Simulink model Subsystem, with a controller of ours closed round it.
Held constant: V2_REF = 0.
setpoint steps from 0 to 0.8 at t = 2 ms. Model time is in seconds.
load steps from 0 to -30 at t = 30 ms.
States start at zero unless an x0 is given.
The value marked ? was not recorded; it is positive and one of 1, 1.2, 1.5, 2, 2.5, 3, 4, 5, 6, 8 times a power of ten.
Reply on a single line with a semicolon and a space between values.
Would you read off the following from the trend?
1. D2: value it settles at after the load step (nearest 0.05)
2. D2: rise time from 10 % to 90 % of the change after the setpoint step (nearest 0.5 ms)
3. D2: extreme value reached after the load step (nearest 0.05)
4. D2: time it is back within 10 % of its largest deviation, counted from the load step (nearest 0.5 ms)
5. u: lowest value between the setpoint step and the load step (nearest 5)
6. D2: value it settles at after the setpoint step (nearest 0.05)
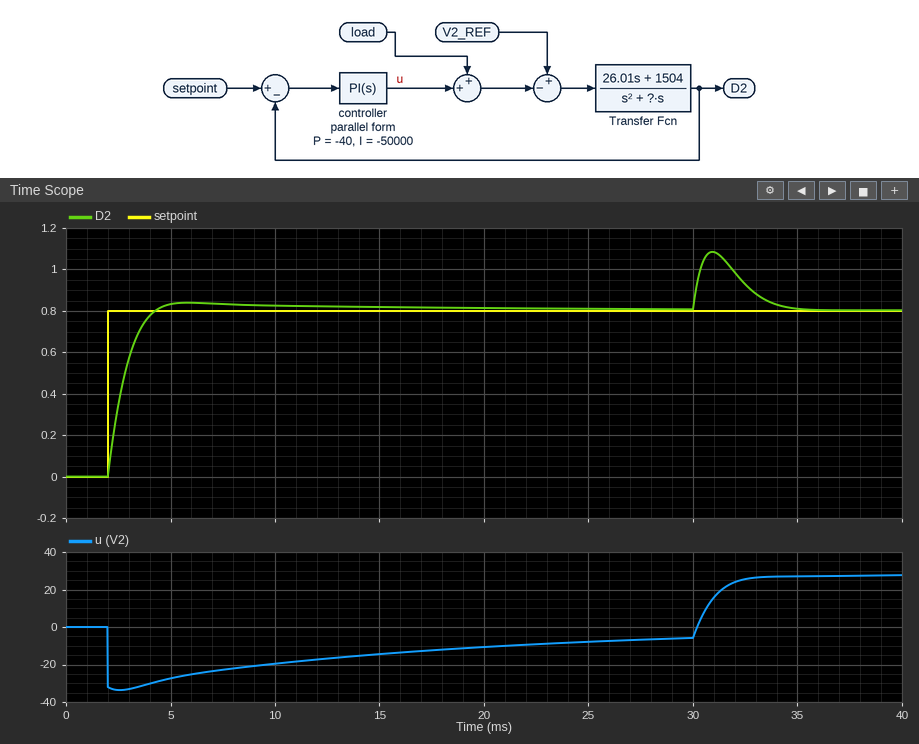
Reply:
0.80; 1.5 ms; 1.10; 4.0 ms; -35; 0.80
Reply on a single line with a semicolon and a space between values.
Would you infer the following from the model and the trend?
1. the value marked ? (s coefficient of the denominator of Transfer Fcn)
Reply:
1000
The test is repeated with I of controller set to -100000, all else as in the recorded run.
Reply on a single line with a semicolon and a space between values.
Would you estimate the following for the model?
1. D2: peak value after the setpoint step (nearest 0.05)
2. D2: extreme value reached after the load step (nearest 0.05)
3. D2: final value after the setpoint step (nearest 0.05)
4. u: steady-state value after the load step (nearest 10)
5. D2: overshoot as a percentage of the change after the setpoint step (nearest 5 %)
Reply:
0.90; 1.05; 0.80; 30; 15 %
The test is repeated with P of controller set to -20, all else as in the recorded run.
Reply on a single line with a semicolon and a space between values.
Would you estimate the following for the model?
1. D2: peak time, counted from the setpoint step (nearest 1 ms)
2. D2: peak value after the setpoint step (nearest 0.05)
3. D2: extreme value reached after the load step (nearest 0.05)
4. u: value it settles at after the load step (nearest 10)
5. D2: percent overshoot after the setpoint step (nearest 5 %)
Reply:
3 ms; 0.90; 1.15; 30; 10 %
